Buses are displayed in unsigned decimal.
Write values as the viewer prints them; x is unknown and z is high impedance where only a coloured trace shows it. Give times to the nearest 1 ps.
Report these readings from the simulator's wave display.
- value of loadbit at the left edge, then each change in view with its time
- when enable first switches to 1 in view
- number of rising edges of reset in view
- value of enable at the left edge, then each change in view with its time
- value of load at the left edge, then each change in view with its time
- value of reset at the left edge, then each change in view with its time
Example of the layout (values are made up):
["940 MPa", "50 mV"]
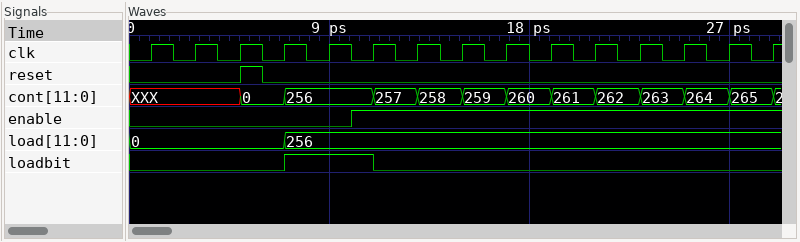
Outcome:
["0, 1 at 7 ps, 0 at 11 ps", "10 ps", "1", "0, 1 at 10 ps", "0, 256 at 7 ps", "0, 1 at 5 ps, 0 at 6 ps"]
